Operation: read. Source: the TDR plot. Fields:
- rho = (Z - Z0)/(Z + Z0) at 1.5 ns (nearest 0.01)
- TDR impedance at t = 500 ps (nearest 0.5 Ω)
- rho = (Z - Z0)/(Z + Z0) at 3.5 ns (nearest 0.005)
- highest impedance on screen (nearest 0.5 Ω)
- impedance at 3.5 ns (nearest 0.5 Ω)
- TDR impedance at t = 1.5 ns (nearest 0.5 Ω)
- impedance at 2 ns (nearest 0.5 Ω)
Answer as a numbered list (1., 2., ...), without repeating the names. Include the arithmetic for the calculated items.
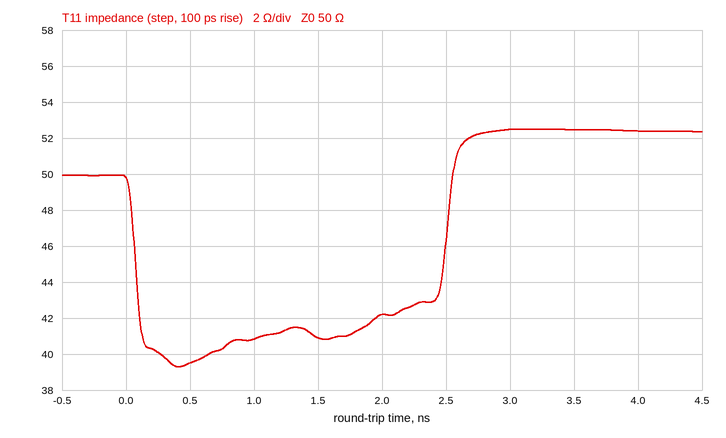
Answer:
1. (41 − 50)/(41 + 50) ≈ -0.10
2. 39.5 Ω
3. (52.5 − 50)/(52.5 + 50) ≈ +0.0244, so +0.025 to the nearest 0.005
4. 52.5 Ω
5. 52.5 Ω
6. 41.0 Ω
7. 42.0 Ω
